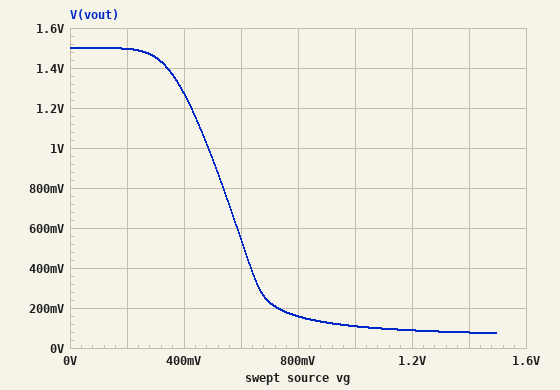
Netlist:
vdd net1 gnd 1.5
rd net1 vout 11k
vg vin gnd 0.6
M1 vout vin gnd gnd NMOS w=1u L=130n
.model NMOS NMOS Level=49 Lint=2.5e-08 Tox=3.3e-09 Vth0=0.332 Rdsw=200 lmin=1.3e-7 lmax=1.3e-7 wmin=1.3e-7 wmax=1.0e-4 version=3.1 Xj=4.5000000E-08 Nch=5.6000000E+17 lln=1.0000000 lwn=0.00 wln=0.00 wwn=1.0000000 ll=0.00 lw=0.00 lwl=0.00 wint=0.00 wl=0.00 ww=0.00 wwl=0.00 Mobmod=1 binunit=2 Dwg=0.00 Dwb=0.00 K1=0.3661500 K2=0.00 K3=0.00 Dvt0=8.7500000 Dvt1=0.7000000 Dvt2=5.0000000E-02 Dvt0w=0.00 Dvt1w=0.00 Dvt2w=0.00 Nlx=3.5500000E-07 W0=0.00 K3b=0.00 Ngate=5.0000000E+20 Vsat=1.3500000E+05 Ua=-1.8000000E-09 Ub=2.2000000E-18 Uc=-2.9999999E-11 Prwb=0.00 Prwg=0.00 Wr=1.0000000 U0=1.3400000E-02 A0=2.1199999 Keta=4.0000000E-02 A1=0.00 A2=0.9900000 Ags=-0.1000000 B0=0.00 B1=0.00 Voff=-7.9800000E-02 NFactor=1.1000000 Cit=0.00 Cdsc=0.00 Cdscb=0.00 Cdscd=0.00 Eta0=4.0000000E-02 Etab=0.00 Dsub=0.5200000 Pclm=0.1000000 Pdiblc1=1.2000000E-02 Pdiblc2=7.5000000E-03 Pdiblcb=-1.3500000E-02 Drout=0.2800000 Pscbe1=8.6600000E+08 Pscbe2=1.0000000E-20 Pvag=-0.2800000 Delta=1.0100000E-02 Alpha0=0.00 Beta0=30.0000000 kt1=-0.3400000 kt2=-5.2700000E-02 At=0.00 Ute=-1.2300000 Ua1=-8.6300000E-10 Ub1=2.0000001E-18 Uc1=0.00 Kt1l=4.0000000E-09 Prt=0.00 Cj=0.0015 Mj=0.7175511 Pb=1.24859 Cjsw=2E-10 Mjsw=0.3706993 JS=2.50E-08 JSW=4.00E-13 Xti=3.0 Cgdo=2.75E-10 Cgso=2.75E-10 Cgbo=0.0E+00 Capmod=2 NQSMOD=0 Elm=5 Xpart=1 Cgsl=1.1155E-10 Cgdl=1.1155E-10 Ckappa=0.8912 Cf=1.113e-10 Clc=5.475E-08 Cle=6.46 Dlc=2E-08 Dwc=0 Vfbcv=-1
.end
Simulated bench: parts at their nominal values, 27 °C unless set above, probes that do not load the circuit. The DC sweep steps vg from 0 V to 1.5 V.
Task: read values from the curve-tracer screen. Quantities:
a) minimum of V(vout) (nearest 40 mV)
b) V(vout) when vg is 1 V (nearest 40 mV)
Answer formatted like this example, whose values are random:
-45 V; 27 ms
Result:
80 mV; 120 mV
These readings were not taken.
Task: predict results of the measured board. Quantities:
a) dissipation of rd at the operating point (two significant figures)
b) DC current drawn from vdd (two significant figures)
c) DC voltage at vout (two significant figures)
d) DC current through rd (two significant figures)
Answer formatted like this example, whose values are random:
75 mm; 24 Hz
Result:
83 µW; 87 µA; 540 mV; 87 µA
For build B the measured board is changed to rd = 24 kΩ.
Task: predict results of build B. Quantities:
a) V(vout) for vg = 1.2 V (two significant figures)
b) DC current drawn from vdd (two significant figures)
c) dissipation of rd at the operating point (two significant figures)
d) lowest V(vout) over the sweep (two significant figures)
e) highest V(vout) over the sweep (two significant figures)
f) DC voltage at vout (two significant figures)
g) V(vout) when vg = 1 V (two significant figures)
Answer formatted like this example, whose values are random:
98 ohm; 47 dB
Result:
40 mV; 57 µA; 78 µW; 34 mV; 1.5 V; 130 mV; 48 mV
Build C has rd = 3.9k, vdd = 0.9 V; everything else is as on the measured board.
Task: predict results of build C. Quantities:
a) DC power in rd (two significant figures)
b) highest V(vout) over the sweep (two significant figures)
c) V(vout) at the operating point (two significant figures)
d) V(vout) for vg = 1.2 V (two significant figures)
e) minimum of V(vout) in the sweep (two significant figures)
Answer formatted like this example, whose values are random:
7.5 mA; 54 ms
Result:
30 µW; 900 mV; 560 mV; 140 mV; 120 mV
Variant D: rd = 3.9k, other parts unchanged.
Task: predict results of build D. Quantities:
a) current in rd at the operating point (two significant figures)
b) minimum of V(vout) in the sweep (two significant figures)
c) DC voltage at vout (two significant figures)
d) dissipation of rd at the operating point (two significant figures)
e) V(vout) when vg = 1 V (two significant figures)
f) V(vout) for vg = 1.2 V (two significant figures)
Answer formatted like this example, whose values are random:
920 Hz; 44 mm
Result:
100 µA; 210 mV; 1.1 V; 39 µW; 360 mV; 270 mV
